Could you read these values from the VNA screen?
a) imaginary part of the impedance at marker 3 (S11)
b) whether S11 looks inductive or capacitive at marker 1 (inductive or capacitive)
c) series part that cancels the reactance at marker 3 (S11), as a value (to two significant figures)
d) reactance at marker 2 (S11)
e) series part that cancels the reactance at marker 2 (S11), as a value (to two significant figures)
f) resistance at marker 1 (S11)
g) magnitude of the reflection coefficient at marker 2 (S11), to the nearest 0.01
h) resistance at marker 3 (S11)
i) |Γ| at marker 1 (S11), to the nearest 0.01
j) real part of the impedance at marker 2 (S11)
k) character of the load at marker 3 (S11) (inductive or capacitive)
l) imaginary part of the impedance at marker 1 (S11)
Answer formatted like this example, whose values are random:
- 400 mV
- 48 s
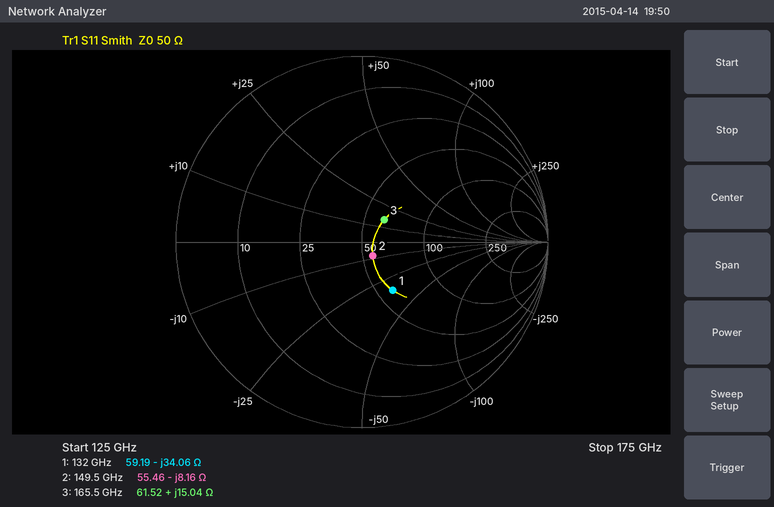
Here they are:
- +15.04 Ω
- capacitive
- 64 fF
- -8.16 Ω
- 8.7 pH
- 59.19 Ω
- 0.09
- 61.52 Ω
- 0.31
- 55.46 Ω
- inductive
- -34.06 Ω
